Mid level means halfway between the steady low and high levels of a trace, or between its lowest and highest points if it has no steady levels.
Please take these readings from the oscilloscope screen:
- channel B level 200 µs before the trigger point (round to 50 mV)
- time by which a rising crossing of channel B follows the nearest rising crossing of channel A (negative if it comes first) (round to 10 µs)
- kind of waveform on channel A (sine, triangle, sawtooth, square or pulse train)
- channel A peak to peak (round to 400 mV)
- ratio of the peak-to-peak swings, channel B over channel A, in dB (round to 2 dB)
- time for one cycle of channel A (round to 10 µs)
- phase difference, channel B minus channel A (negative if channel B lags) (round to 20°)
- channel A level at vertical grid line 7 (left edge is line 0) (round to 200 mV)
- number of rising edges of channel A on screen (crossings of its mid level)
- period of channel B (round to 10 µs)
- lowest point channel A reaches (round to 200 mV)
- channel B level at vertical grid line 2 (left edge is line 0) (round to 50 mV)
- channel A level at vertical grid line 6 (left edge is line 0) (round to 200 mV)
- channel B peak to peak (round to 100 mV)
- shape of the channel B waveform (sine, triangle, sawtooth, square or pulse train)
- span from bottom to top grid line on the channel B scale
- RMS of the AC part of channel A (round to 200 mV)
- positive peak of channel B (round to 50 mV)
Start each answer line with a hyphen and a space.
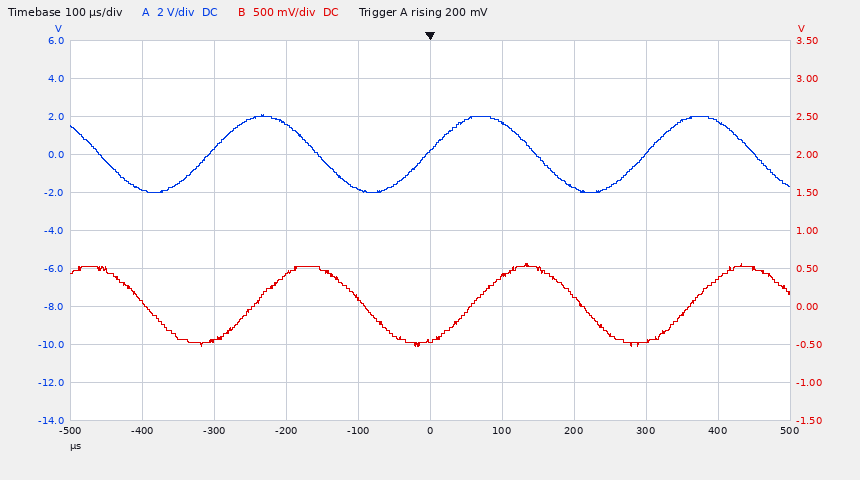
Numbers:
- 450 mV
- +60 µs
- sine
- 4.0 V
- -12 dB
- 300 µs
- -80°
- -1.8 V
- 3
- 300 µs
- -2.0 V
- -450 mV
- 1.6 V
- 1.10 V
- sine
- 5 V
- 1.4 V
- 550 mV
